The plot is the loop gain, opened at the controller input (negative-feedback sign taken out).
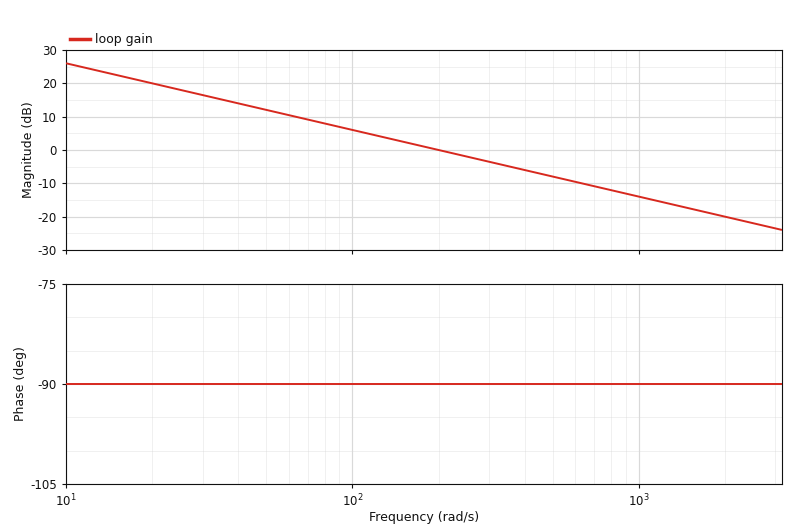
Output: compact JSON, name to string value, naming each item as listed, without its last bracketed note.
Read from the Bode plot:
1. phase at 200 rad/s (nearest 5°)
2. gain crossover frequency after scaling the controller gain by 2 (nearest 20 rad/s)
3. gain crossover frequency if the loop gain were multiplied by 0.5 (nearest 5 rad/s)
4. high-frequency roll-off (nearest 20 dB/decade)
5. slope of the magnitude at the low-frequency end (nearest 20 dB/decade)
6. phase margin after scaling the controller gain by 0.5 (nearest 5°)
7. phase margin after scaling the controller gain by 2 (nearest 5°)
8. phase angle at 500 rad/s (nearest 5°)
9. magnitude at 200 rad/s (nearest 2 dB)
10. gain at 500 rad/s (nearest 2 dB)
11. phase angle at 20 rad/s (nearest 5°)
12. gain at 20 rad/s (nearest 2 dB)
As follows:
{"phase at 200 rad/s": "-90°", "gain crossover frequency after scaling the controller gain by 2": "400 rad/s", "gain crossover frequency if the loop gain were multiplied by 0.5": "100 rad/s", "high-frequency roll-off": "-20 dB/decade", "slope of the magnitude at the low-frequency end": "-20 dB/decade", "phase margin after scaling the controller gain by 0.5": "90°", "phase margin after scaling the controller gain by 2": "90°", "phase angle at 500 rad/s": "-90°", "magnitude at 200 rad/s": "0 dB", "gain at 500 rad/s": "-8 dB", "phase angle at 20 rad/s": "-90°", "gain at 20 rad/s": "20 dB"}
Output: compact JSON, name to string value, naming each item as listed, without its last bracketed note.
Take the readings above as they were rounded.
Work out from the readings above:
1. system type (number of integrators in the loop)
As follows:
{"system type": "1"}
